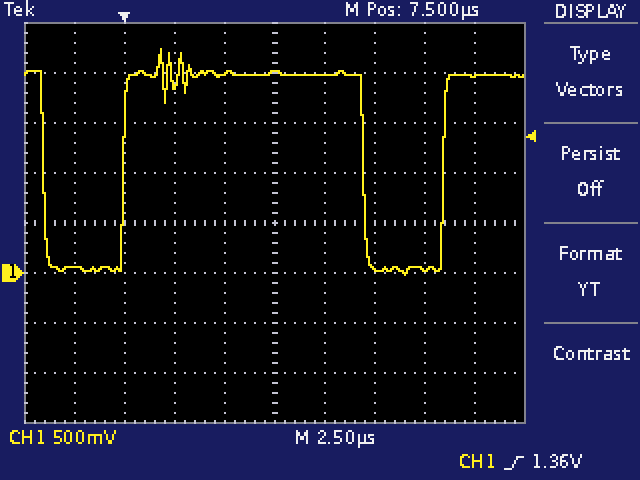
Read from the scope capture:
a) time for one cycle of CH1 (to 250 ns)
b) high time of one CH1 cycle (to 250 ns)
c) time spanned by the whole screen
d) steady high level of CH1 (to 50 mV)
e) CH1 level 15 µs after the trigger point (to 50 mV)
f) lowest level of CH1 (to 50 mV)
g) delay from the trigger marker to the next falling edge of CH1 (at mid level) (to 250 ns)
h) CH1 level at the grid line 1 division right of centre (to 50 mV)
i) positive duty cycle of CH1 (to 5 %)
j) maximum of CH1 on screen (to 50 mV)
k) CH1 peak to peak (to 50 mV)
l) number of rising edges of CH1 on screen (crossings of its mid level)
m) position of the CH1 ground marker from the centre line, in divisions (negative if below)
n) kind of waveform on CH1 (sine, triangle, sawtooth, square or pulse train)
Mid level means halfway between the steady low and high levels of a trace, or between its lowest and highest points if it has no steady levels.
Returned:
16.00 µs
12.00 µs
25 µs
2.00 V
50 mV
0 mV
12.00 µs
2.00 V
75 %
2.25 V
2.25 V
2
-1.0 div
pulse train
